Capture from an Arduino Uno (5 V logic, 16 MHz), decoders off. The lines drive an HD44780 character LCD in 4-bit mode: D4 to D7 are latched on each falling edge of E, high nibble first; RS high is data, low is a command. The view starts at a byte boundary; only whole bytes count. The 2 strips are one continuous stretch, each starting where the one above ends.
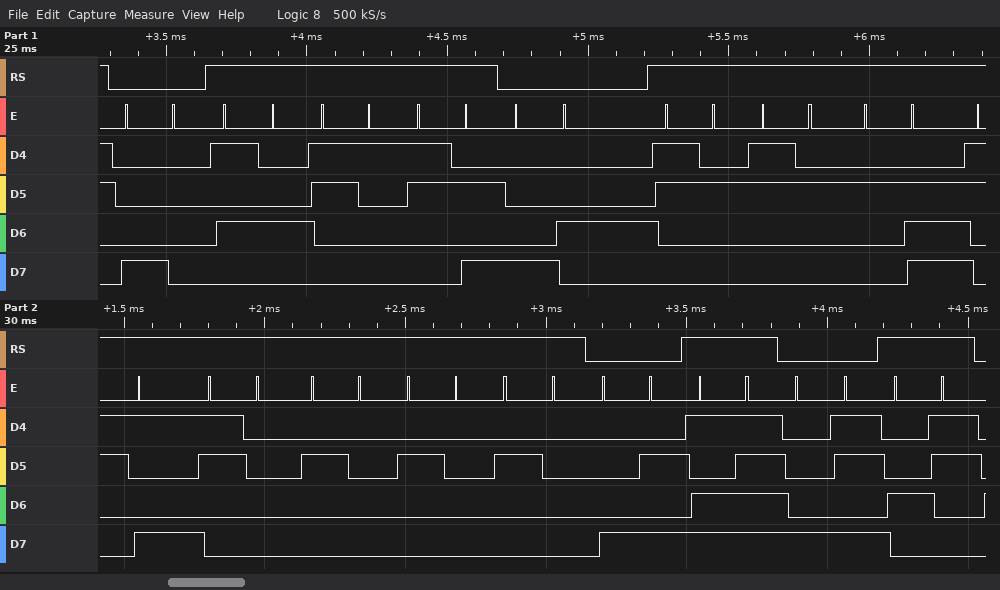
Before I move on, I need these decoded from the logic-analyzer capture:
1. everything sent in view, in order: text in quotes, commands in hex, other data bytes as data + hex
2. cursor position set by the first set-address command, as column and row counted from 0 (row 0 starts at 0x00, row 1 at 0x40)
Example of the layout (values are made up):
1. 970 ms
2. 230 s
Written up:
1. 0x80 "T1:" 0x84 "22.90   " 0x8A data DF 0x8B "C"
2. column 0, row 0
